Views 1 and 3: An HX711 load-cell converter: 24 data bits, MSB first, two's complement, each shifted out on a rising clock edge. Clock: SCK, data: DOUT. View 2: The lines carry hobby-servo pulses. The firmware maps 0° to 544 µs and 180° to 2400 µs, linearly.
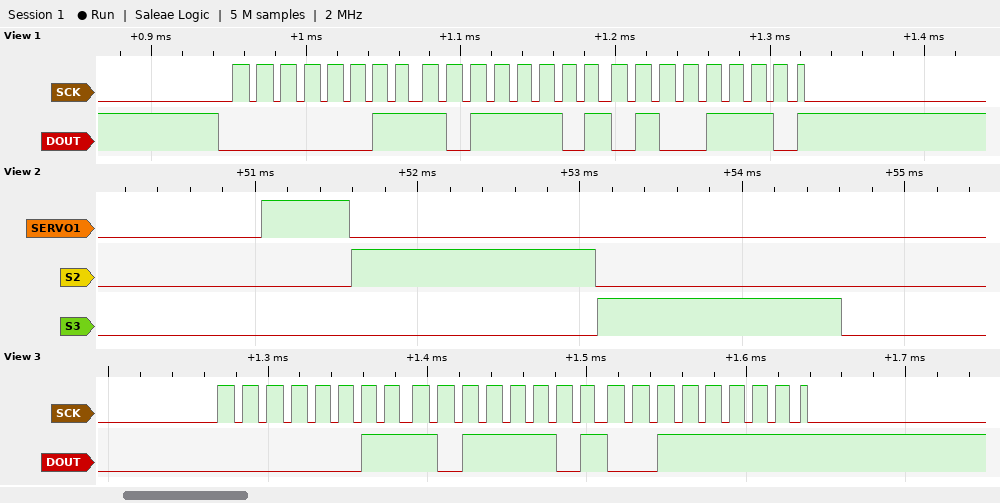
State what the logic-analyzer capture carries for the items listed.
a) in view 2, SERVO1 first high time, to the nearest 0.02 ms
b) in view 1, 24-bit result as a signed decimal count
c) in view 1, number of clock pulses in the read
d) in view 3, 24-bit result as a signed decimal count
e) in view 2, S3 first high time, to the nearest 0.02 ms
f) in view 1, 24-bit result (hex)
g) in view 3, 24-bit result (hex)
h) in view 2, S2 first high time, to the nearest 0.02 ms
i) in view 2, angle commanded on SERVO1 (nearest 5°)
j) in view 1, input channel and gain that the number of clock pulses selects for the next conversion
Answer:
0.54 ms
245070
25
245055
1.50 ms
0x03BD4E
0x03BD3F
1.50 ms
0°
channel A, gain 128
